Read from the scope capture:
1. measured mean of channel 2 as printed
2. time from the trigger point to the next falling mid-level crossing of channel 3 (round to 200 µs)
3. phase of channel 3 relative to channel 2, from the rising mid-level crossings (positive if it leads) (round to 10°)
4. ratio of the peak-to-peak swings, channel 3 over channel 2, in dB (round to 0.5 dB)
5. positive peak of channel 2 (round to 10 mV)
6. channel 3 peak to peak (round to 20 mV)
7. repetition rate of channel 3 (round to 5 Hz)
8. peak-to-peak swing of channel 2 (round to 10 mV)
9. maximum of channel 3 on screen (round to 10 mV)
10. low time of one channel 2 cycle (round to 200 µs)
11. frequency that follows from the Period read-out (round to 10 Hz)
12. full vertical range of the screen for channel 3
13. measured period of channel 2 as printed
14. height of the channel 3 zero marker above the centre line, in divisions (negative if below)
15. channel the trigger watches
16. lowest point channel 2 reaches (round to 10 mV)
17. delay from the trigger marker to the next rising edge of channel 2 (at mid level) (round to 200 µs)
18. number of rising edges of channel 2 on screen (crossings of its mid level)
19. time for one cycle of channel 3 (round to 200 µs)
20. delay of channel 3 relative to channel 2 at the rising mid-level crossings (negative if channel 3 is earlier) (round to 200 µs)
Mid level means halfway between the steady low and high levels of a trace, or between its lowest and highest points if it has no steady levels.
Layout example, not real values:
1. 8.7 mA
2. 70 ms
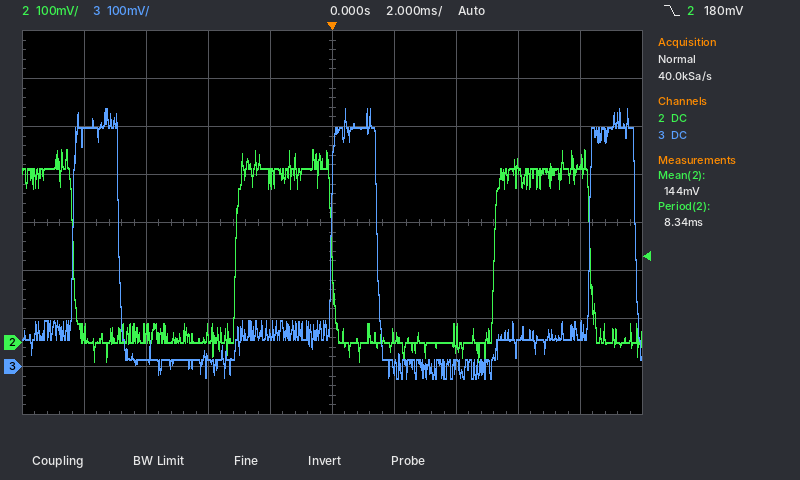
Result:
1. 144 mV
2. 1.4 ms
3. -130°
4. 2.0 dB
5. 400 mV
6. 560 mV
7. 120 Hz
8. 440 mV
9. 540 mV
10. 5.2 ms
11. 120 Hz
12. 800 mV
13. 8.34 ms
14. -3.0 div
15. channel 2
16. -40 mV
17. 5.2 ms
18. 2
19. 8.4 ms
20. +3.0 ms
